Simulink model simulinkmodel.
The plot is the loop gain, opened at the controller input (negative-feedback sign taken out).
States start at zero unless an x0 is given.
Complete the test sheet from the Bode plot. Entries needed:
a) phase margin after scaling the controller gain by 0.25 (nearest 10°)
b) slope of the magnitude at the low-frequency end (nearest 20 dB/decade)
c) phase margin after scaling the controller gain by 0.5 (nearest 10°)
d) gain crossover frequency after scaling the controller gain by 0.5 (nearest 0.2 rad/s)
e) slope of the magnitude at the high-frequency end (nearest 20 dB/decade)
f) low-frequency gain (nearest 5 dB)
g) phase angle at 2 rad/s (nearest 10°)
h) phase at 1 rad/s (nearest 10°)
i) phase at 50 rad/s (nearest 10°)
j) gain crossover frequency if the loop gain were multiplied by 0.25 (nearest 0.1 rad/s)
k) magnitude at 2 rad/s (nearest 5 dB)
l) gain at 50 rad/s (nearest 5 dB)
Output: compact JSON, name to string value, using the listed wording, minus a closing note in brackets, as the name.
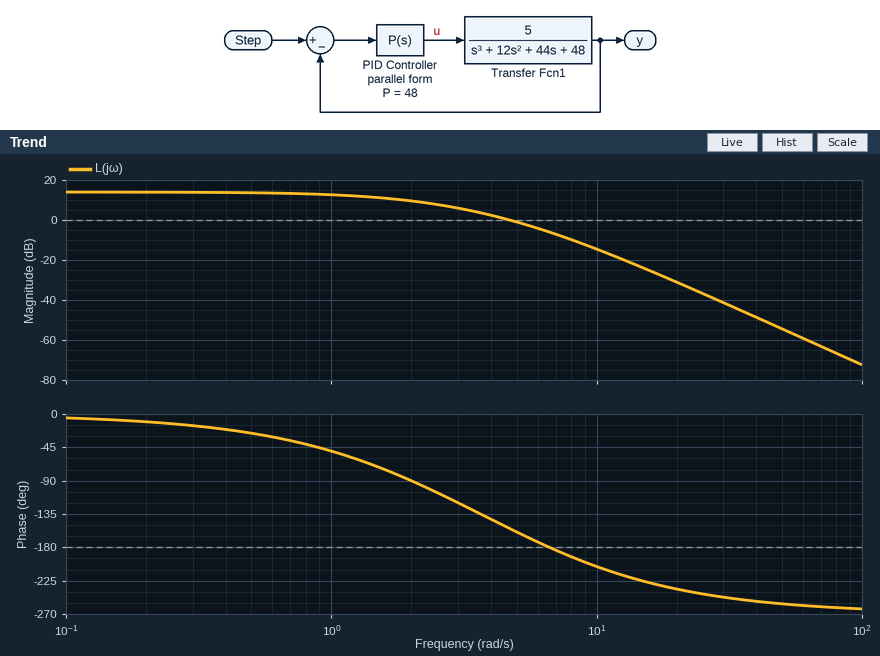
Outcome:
{"phase margin after scaling the controller gain by 0.25": "120°", "slope of the magnitude at the low-frequency end": "0 dB/decade", "phase margin after scaling the controller gain by 0.5": "60°", "gain crossover frequency after scaling the controller gain by 0.5": "3.0 rad/s", "slope of the magnitude at the high-frequency end": "-60 dB/decade", "low-frequency gain": "15 dB", "phase angle at 2 rad/s": "-90°", "phase at 1 rad/s": "-50°", "phase at 50 rad/s": "-260°", "gain crossover frequency if the loop gain were multiplied by 0.25": "1.2 rad/s", "magnitude at 2 rad/s": "10 dB", "gain at 50 rad/s": "-55 dB"}
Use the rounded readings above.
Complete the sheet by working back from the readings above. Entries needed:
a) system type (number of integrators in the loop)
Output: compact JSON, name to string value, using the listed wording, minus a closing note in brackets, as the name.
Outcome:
{"system type": "0"}
